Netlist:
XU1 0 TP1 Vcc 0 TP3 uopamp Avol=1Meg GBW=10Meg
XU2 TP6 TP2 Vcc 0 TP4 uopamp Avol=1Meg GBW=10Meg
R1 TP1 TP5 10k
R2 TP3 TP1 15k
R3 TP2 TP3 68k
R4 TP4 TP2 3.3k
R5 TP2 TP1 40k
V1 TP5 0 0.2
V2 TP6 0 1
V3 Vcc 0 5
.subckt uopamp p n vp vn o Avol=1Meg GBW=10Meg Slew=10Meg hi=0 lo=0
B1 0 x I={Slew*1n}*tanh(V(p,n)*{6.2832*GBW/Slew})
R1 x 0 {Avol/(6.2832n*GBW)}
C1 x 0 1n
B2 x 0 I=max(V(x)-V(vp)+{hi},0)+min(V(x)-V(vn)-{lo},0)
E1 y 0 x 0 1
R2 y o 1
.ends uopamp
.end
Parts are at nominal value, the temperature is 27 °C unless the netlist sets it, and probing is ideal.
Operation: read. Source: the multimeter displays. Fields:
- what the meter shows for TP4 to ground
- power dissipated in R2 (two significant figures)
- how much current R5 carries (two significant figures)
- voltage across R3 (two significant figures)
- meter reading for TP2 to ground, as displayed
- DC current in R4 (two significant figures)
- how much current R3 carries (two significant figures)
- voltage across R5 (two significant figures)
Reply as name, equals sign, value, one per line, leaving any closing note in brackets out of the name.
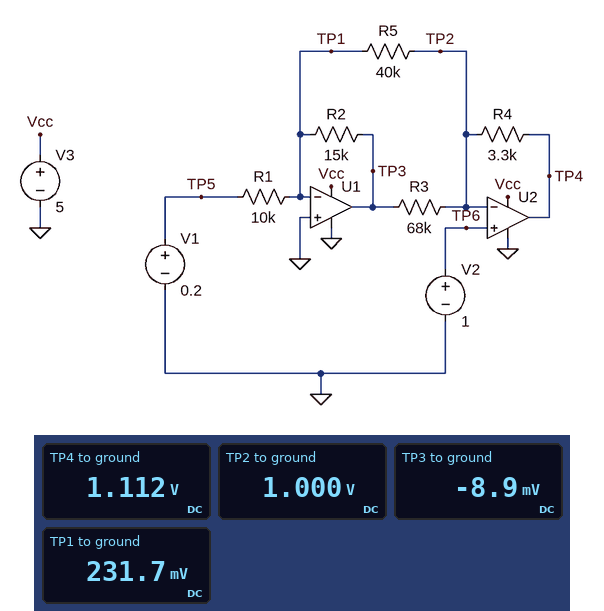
what the meter shows for TP4 to ground = 1.112 V
power dissipated in R2 = 3.9 µW
how much current R5 carries = 19 µA
voltage across R3 = 1.0 V
meter reading for TP2 to ground, as displayed = 1.000 V
DC current in R4 = 34 µA
how much current R3 carries = 15 µA
voltage across R5 = 770 mV
